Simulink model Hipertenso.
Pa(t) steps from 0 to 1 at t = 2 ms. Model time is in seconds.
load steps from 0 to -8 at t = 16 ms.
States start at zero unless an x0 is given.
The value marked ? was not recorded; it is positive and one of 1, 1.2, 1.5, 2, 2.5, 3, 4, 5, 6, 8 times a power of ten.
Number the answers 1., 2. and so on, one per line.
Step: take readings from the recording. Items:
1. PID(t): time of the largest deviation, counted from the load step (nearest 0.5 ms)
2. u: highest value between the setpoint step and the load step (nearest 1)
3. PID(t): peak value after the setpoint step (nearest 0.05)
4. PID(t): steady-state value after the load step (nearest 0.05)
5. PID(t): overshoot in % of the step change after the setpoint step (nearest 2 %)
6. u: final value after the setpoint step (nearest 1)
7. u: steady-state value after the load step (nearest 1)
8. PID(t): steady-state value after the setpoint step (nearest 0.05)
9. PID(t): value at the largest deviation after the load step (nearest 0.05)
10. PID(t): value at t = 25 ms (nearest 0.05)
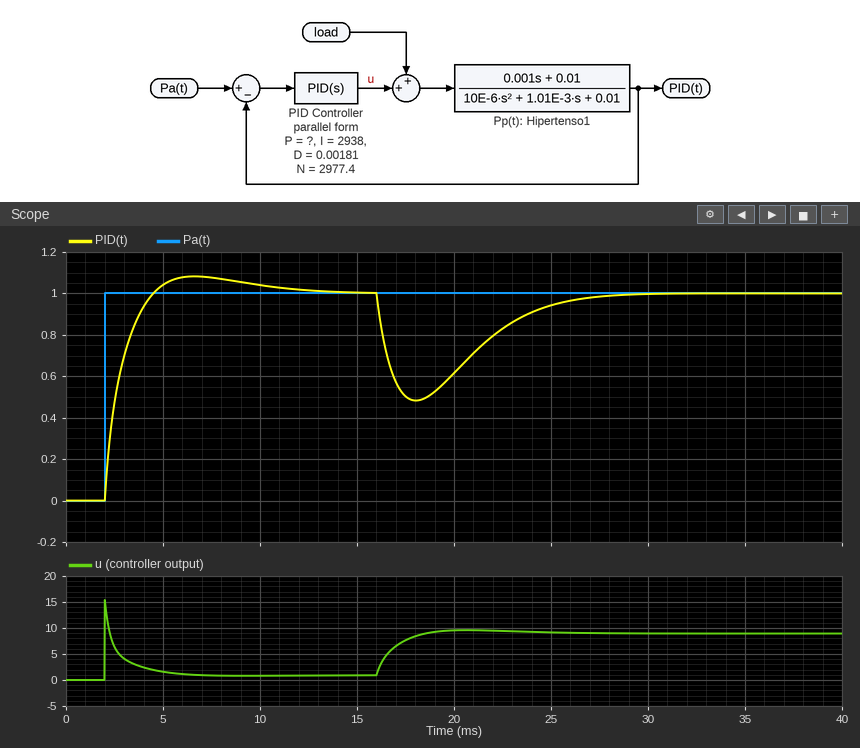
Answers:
1. 2.0 ms
2. 15
3. 1.10
4. 1.00
5. 8 %
6. 1
7. 9
8. 1.00
9. 0.50
10. 0.95
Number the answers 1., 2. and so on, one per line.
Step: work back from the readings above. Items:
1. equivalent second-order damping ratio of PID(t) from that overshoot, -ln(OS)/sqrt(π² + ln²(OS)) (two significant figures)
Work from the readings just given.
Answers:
1. 0.63
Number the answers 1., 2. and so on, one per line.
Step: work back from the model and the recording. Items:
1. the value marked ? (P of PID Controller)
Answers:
1. 10
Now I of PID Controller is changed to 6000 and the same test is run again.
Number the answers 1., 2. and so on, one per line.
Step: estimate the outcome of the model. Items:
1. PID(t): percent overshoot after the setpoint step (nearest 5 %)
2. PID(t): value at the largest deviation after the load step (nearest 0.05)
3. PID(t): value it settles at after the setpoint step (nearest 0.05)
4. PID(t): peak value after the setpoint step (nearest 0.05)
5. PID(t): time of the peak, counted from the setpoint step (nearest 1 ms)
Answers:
1. 15 %
2. 0.55
3. 1.00
4. 1.15
5. 3 ms
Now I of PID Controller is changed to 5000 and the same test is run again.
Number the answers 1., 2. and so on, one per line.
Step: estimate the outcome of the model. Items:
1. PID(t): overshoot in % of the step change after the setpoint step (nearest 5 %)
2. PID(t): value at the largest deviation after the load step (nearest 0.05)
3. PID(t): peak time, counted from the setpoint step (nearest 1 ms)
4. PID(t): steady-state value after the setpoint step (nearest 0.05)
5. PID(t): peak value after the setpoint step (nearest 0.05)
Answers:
1. 15 %
2. 0.55
3. 4 ms
4. 1.00
5. 1.15
